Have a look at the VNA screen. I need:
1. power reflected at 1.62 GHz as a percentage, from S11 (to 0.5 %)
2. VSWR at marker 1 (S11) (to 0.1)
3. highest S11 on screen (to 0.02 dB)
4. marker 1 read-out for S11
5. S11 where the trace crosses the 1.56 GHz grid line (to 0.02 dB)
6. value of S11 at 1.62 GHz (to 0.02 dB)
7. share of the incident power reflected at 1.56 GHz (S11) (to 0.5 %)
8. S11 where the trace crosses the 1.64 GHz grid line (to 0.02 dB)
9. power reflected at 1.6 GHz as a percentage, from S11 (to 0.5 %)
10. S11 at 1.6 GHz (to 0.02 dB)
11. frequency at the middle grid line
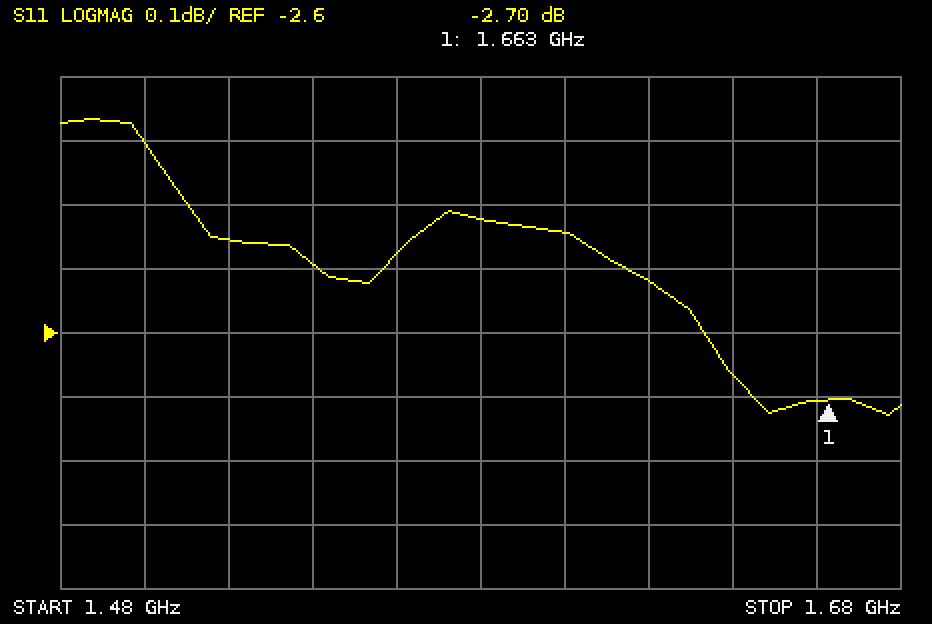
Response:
56.0 %
6.5
-2.26 dB
-2.70 dB
-2.48 dB
-2.52 dB
56.5 %
-2.66 dB
57.0 %
-2.44 dB
1.58 GHz
